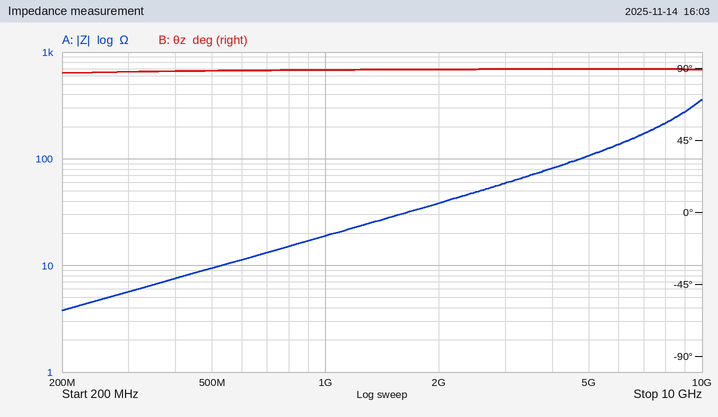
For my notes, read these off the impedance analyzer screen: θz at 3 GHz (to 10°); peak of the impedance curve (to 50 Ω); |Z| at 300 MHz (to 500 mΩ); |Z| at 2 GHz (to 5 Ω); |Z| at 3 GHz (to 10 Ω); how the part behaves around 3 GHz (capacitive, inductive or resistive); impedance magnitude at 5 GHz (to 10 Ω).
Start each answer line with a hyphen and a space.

- 90°
- 350 Ω
- 5.5 Ω
- 40 Ω
- 60 Ω
- inductive
- 110 Ω
